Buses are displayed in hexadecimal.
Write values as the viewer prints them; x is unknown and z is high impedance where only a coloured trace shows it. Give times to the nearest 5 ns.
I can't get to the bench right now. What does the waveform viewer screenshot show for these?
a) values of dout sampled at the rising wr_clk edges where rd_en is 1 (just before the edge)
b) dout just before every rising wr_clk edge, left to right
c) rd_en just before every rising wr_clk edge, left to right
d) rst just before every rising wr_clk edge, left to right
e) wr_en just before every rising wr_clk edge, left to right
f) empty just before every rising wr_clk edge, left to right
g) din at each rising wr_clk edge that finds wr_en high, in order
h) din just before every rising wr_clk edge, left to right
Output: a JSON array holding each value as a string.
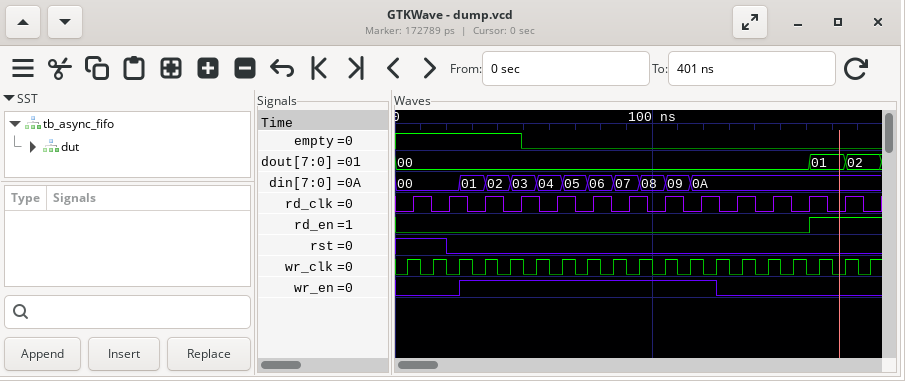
["01, 01, 02", "00, 00, 00, 00, 00, 00, 00, 00, 00, 00, 00, 00, 00, 00, 00, 00, 01, 01, 02", "0 0 0 0 0 0 0 0 0 0 0 0 0 0 0 0 1 1 1", "1 1 0 0 0 0 0 0 0 0 0 0 0 0 0 0 0 0 0", "0 0 0 1 1 1 1 1 1 1 1 1 1 0 0 0 0 0 0", "1 1 1 1 1 0 0 0 0 0 0 0 0 0 0 0 0 0 0", "01, 02, 03, 04, 05, 06, 07, 08, 09, 0A", "00, 00, 00, 01, 02, 03, 04, 05, 06, 07, 08, 09, 0A, 0A, 0A, 0A, 0A, 0A, 0A"]
